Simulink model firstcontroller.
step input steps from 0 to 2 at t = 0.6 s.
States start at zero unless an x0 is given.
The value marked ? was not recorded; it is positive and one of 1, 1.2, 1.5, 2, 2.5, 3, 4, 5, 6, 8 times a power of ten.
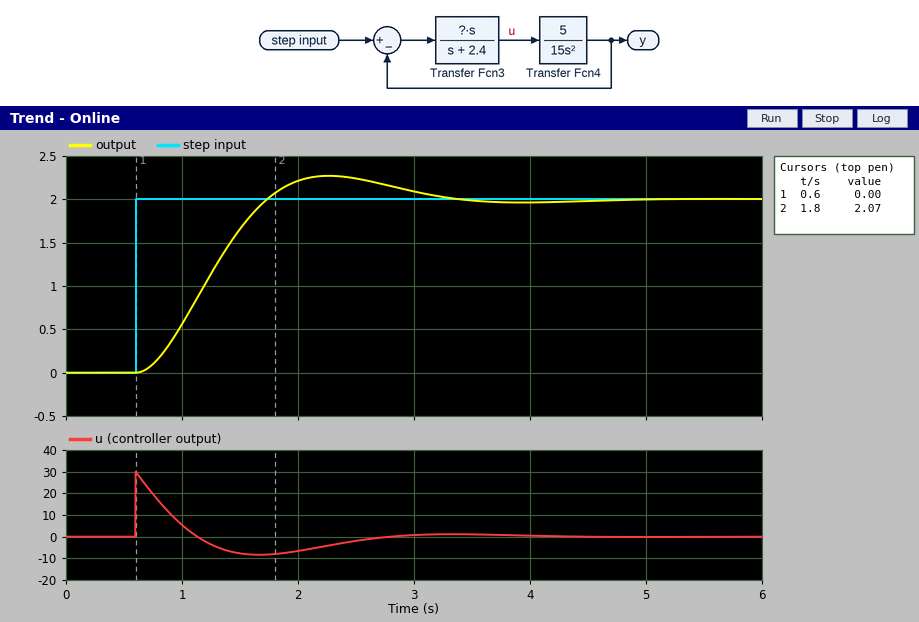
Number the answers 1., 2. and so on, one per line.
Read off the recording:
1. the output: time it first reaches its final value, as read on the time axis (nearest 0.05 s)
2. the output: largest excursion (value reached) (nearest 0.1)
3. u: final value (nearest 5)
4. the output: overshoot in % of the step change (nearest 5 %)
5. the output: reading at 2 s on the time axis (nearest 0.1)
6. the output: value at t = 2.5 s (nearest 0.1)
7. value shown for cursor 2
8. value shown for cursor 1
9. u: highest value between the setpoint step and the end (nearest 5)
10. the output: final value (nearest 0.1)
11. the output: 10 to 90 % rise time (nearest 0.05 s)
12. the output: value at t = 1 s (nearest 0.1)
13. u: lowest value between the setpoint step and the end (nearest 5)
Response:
1. 1.75 s
2. 2.3
3. 0
4. 15 %
5. 2.2
6. 2.2
7. 2.07
8. 0.00
9. 30
10. 2.0
11. 0.75 s
12. 0.6
13. -10
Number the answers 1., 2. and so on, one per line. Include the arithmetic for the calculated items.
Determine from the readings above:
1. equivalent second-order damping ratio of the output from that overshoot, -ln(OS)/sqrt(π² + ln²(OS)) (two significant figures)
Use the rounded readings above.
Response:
1. ln(0.15) = -1.897; 1.897 / sqrt(9.870 + 3.599) = 0.52
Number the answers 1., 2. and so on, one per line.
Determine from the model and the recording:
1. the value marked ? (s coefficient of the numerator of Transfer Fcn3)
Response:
1. 15
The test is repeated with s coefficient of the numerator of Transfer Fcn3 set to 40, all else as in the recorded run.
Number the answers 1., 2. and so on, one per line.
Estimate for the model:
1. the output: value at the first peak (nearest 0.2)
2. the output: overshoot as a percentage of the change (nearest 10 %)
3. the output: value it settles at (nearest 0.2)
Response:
1. 2.6
2. 30 %
3. 2.0
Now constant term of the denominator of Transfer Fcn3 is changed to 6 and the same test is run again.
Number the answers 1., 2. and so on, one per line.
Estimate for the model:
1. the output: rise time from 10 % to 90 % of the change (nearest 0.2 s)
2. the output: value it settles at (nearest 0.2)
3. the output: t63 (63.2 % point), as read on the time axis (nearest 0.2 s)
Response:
1. 2.2 s
2. 2.0
3. 1.8 s
